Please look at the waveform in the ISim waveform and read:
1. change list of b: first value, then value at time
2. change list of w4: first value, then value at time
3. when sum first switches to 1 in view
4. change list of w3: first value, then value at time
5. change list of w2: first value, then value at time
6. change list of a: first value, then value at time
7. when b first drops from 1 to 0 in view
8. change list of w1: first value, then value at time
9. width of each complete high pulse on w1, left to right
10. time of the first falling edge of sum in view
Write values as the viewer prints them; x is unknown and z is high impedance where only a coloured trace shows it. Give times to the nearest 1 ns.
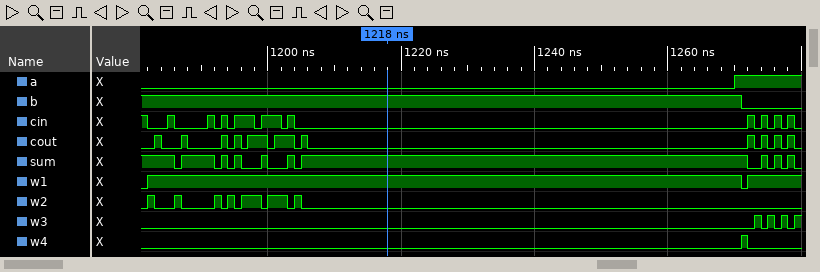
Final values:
1, 0 at 1271 ns
0, 1 at 1271 ns, 0 at 1272 ns
1187 ns
0, 1 at 1273 ns, 0 at 1274 ns, 1 at 1275 ns, 0 at 1276 ns, 1 at 1277 ns, 0 at 1278 ns, 1 at 1279 ns
0, 1 at 1182 ns, 0 at 1183 ns, 1 at 1186 ns, 0 at 1187 ns, 1 at 1192 ns, 0 at 1193 ns, 1 at 1194 ns, 0 at 1195 ns, 1 at 1196 ns, 0 at 1199 ns, 1 at 1200 ns, 0 at 1203 ns, 1 at 1204 ns, 0 at 1205 ns
0, 1 at 1270 ns
1271 ns
0, 1 at 1182 ns, 0 at 1271 ns, 1 at 1272 ns
89 ns
1186 ns
